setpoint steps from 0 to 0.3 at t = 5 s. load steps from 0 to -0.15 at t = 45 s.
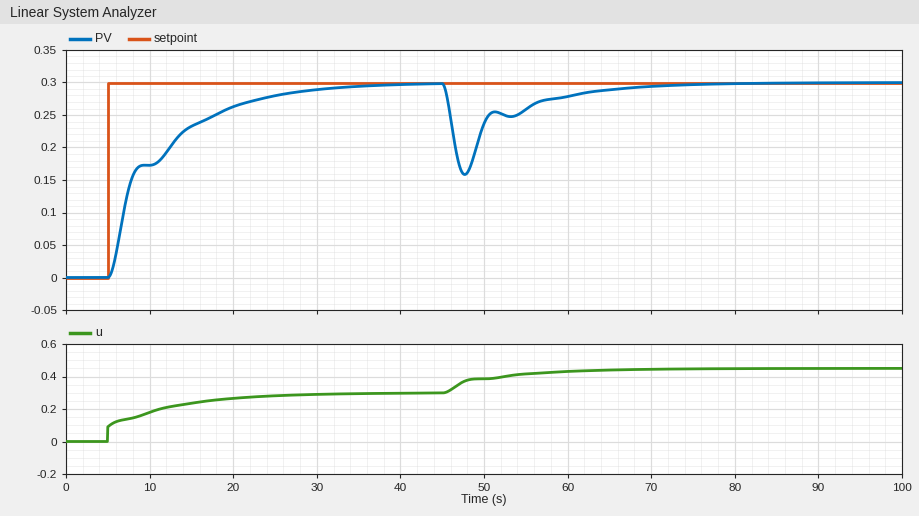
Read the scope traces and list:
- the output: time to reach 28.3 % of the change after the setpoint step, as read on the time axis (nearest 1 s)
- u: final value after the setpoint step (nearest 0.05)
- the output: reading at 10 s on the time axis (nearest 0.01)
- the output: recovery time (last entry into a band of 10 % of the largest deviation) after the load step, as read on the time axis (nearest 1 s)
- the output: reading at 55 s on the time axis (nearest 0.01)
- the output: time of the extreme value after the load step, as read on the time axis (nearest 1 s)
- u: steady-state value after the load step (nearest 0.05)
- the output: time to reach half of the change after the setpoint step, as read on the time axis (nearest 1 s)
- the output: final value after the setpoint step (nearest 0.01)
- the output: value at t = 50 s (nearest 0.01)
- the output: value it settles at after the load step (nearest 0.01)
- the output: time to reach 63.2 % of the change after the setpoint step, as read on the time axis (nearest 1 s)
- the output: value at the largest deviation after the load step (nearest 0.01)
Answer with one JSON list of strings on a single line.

["7 s", "0.30", "0.17", "63 s", "0.26", "48 s", "0.45", "8 s", "0.30", "0.24", "0.30", "12 s", "0.16"]
